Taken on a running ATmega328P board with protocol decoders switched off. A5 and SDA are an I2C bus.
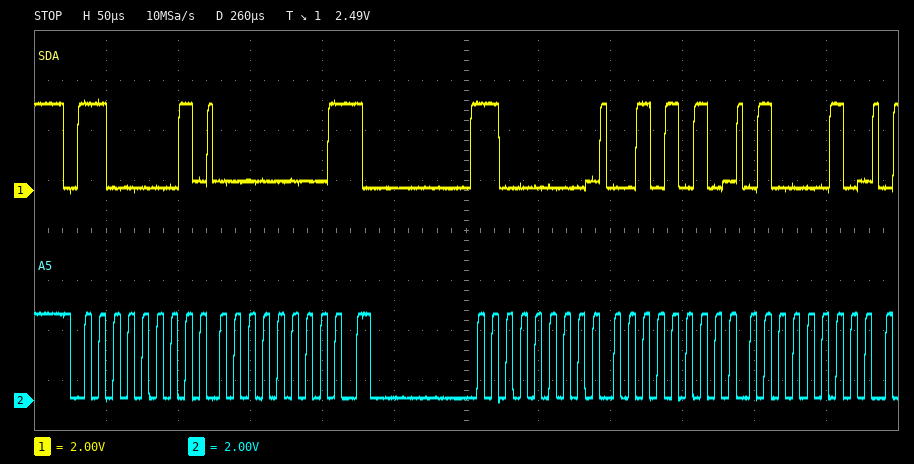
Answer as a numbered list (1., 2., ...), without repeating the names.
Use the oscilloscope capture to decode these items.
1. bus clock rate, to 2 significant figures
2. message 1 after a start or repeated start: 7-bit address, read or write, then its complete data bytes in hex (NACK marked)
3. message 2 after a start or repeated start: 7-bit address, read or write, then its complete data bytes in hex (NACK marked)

1. 100 kHz
2. 0x60 read: 00 NACK
3. 0x60 write: 2A 42
